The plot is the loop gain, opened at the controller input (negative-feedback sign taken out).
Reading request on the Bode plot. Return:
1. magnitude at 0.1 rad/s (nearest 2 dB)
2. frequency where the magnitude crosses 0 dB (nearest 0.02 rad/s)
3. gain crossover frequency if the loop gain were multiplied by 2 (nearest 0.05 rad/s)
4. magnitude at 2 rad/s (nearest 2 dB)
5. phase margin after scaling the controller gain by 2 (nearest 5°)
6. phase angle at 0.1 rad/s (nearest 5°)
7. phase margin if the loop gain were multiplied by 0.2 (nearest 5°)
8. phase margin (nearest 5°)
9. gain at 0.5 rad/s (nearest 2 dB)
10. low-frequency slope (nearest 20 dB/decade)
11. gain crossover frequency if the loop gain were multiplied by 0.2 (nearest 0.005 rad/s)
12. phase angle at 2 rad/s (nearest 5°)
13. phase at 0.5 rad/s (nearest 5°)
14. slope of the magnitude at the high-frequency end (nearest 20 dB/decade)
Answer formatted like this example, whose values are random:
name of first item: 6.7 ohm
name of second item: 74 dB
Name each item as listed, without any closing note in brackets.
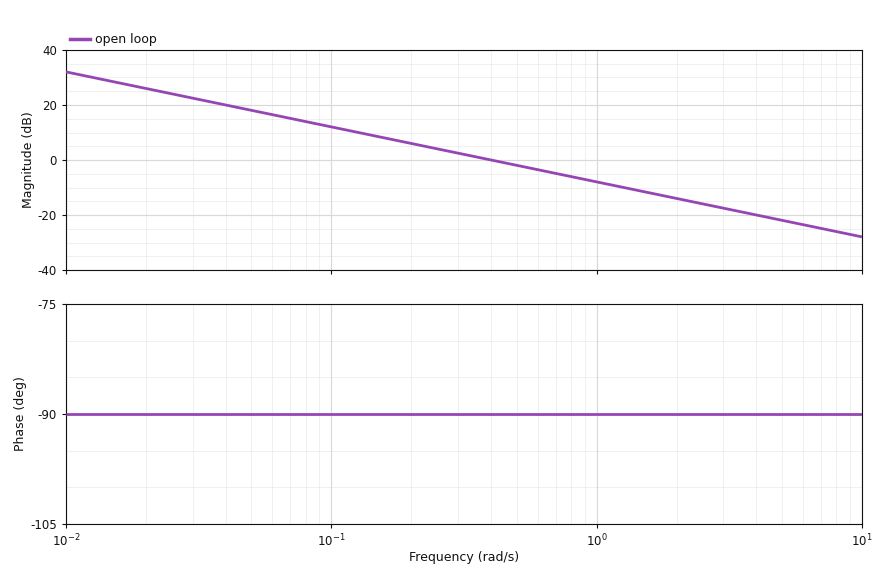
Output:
magnitude at 0.1 rad/s: 12 dB
frequency where the magnitude crosses 0 dB: 0.40 rad/s
gain crossover frequency if the loop gain were multiplied by 2: 0.80 rad/s
magnitude at 2 rad/s: -14 dB
phase margin after scaling the controller gain by 2: 90°
phase angle at 0.1 rad/s: -90°
phase margin if the loop gain were multiplied by 0.2: 90°
phase margin: 90°
gain at 0.5 rad/s: -2 dB
low-frequency slope: -20 dB/decade
gain crossover frequency if the loop gain were multiplied by 0.2: 0.080 rad/s
phase angle at 2 rad/s: -90°
phase at 0.5 rad/s: -90°
slope of the magnitude at the high-frequency end: -20 dB/decade
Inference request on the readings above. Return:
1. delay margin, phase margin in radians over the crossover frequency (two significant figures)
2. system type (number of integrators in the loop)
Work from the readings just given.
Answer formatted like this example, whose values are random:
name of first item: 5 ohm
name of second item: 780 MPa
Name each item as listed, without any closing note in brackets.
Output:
delay margin, phase margin in radians over the crossover frequency: 3.9 s
system type: 1
